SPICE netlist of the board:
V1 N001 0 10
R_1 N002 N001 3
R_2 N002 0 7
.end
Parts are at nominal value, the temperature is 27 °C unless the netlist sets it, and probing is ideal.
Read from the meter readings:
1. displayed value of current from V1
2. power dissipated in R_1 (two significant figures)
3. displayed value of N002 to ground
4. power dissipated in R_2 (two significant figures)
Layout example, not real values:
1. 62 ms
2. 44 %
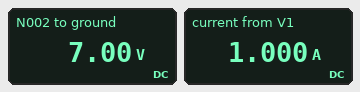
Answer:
1. 1.000 A
2. 3.0 W
3. 7.00 V
4. 7.0 W
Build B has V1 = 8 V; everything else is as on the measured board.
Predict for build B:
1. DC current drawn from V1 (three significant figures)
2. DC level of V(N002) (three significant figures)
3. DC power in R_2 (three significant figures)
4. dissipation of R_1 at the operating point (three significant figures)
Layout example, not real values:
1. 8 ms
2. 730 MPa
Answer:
1. 800 mA
2. 5.60 V
3. 4.48 W
4. 1.92 W
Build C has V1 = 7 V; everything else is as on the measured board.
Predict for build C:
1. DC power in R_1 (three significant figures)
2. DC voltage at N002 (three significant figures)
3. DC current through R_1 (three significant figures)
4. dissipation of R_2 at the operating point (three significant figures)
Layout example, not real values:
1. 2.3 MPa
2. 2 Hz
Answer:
1. 1.47 W
2. 4.90 V
3. 700 mA
4. 3.43 W
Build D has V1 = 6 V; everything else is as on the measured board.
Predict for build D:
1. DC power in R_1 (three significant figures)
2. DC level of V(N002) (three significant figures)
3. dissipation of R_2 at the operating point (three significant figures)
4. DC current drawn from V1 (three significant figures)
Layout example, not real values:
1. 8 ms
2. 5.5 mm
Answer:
1. 1.08 W
2. 4.20 V
3. 2.52 W
4. 600 mA
